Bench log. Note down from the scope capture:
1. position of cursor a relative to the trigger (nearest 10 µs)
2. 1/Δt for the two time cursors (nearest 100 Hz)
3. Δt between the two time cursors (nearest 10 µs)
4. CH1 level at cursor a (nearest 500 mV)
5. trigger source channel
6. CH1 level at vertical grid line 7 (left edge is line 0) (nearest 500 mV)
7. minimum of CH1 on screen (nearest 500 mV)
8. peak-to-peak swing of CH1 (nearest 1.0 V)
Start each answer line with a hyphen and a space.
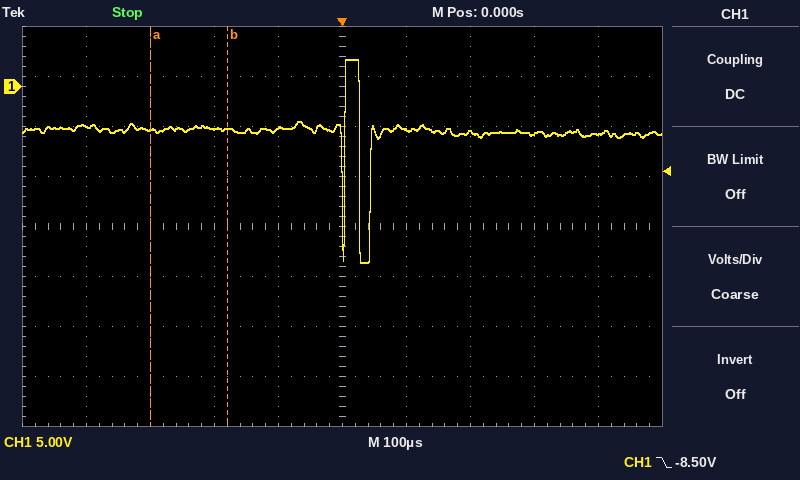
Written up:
- -300 µs
- 8.3 kHz
- 120 µs
- -4.5 V
- CH1
- -4.5 V
- -17.5 V
- 20.0 V
